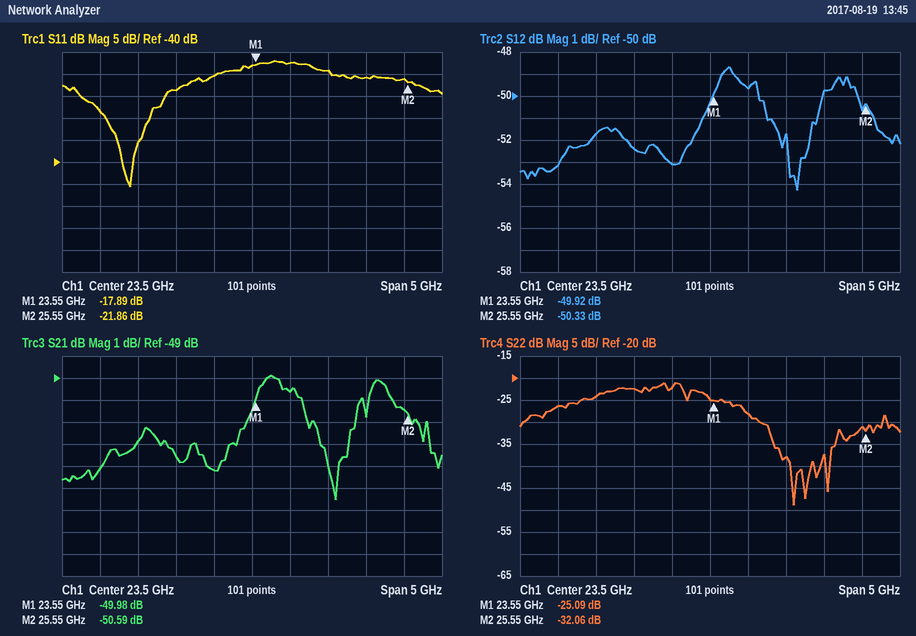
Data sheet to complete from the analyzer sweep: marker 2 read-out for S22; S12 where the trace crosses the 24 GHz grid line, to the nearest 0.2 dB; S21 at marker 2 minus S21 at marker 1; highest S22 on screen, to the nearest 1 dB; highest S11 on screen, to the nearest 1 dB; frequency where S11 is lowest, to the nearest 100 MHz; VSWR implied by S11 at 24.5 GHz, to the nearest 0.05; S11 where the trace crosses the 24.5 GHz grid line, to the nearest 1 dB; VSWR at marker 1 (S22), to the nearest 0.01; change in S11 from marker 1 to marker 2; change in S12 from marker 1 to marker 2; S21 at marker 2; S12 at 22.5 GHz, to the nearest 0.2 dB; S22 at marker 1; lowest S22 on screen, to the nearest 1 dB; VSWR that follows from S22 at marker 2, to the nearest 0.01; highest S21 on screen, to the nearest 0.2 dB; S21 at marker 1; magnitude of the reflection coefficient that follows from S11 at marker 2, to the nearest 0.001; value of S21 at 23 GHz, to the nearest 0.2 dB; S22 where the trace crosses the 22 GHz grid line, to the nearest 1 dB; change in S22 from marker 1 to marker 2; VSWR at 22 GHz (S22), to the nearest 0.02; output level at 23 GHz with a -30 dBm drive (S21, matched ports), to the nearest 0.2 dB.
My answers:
-32.06 dB
-49.6 dB
-0.61 dB
-21 dB
-17 dB
21.9 GHz
1.25
-19 dB
1.12
-3.97 dB
-0.41 dB
-50.59 dB
-52.4 dB
-25.09 dB
-49 dB
1.05
-48.8 dB
-49.98 dB
0.081
-53.2 dB
-24 dB
-6.97 dB
1.14
-83.2 dBm
